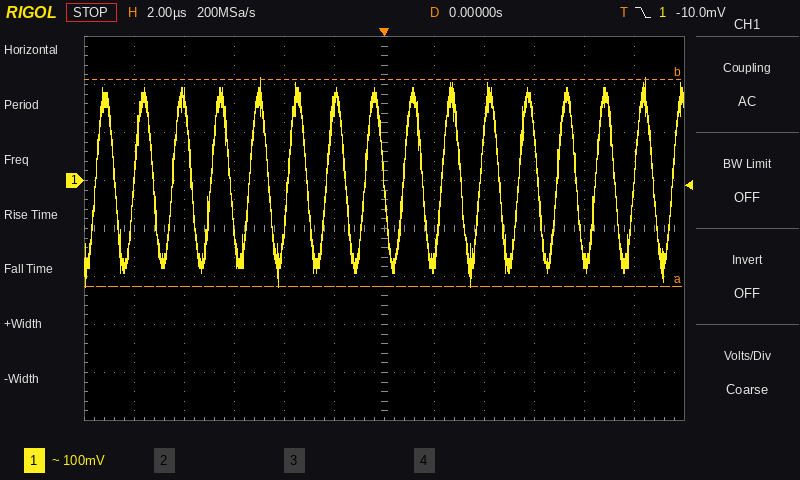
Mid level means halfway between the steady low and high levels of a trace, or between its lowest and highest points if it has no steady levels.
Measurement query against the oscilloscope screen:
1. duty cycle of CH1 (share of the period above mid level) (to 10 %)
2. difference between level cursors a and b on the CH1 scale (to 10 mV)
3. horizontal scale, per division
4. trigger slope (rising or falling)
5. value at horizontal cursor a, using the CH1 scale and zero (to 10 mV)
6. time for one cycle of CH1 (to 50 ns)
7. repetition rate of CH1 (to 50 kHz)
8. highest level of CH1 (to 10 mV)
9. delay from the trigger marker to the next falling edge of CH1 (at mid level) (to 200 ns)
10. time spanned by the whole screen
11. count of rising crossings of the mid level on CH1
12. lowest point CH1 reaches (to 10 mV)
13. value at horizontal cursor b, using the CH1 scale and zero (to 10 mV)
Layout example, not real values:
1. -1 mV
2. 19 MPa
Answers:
1. 50 %
2. 430 mV
3. 2 µs
4. falling
5. -220 mV
6. 1.55 µs
7. 650 kHz
8. 210 mV
9. 1.6 µs
10. 24 µs
11. 16
12. -220 mV
13. 210 mV
